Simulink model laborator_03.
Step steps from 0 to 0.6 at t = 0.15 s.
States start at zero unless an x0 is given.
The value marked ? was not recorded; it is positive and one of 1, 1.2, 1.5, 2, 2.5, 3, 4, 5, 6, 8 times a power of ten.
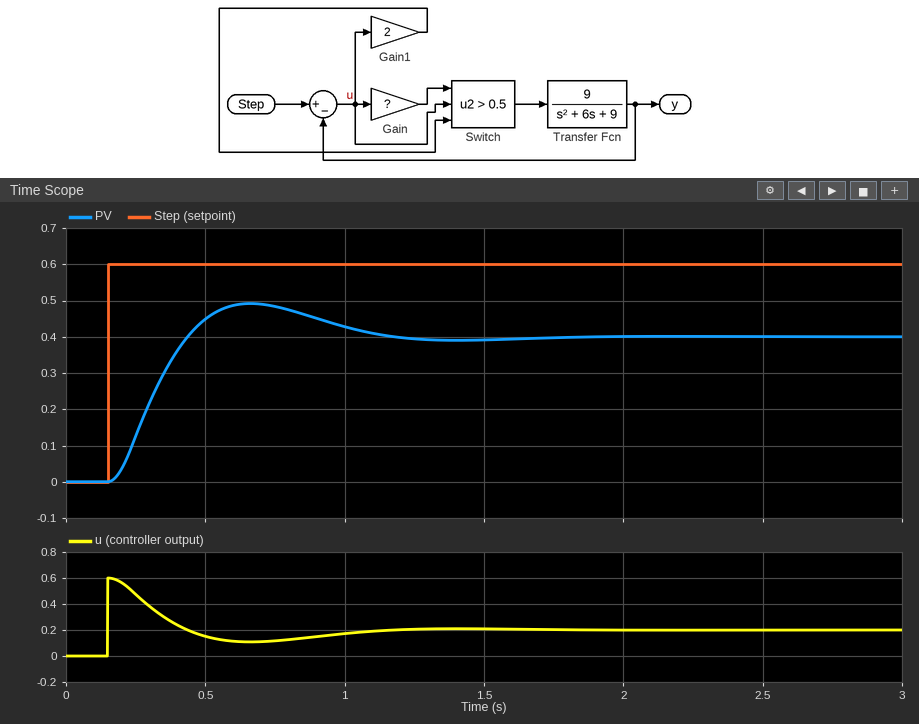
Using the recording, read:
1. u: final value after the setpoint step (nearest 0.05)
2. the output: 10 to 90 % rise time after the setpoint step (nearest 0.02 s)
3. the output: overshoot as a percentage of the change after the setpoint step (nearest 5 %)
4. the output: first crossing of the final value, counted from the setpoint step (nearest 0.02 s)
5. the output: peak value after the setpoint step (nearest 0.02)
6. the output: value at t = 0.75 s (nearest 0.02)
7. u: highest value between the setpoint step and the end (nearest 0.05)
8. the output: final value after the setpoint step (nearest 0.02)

0.20
0.20 s
25 %
0.28 s
0.50
0.48
0.60
0.40
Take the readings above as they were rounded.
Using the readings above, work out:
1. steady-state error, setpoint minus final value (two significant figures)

0.20
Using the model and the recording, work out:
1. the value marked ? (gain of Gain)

6
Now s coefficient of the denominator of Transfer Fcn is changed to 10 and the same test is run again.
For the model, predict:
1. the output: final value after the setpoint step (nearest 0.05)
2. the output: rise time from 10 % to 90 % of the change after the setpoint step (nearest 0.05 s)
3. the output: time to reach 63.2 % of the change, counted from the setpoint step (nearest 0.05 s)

0.40
0.35 s
0.20 s
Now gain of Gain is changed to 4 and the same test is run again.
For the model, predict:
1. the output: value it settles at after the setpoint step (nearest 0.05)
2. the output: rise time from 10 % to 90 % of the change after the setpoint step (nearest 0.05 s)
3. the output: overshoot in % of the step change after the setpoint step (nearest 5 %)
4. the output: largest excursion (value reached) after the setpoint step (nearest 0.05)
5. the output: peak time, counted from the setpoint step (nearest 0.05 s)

0.40
0.25 s
15 %
0.45
0.60 s
